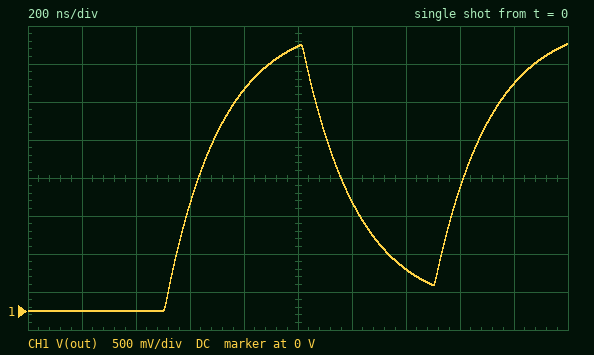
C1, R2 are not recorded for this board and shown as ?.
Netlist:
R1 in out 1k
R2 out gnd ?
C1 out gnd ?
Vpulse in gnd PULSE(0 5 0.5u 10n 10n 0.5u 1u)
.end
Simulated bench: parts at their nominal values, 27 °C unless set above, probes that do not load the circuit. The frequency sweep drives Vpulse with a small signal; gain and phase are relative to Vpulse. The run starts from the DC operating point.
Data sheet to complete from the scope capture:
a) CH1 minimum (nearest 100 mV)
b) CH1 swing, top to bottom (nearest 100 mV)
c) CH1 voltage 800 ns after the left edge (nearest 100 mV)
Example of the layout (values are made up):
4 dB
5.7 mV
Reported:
0 V
3.5 V
2.9 V
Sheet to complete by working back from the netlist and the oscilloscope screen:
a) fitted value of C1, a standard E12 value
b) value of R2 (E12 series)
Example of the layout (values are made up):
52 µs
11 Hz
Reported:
270 pF
3.3 kΩ
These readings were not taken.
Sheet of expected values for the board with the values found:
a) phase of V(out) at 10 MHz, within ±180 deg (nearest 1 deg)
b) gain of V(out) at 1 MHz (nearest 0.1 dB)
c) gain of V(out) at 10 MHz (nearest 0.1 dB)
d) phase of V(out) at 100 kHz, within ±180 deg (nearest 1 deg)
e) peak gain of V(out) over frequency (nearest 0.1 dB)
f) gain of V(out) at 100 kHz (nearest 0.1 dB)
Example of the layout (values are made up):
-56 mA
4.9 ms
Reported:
-86 deg
-6.6 dB
-24.6 dB
-7 deg
-2.3 dB
-2.4 dB
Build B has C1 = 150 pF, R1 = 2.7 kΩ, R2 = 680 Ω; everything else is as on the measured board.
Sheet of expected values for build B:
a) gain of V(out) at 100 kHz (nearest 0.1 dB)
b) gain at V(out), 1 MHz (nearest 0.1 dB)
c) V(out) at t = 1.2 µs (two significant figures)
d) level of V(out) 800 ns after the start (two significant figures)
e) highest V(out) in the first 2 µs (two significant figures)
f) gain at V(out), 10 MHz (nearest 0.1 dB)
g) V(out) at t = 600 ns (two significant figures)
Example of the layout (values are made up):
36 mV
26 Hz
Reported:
-13.9 dB
-14.9 dB
100 mV
980 mV
1.0 V
-28.3 dB
690 mV
